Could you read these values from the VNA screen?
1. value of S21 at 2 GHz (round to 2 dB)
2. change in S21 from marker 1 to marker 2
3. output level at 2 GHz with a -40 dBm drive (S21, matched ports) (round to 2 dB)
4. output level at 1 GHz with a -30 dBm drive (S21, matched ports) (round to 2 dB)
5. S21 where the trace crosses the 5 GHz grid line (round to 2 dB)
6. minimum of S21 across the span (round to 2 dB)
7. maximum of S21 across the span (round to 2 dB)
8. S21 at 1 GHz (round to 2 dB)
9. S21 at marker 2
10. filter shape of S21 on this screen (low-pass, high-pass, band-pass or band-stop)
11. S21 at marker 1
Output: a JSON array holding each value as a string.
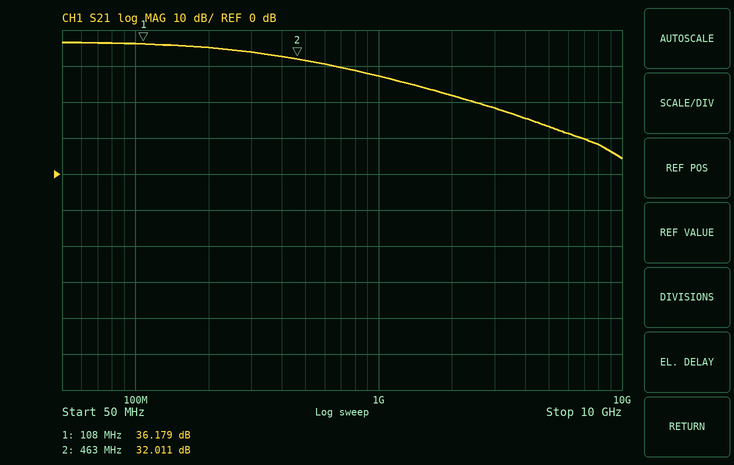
["22 dB", "-4.168 dB", "-18 dBm", "-2 dBm", "14 dB", "4 dB", "36 dB", "28 dB", "32.011 dB", "low-pass", "36.179 dB"]
